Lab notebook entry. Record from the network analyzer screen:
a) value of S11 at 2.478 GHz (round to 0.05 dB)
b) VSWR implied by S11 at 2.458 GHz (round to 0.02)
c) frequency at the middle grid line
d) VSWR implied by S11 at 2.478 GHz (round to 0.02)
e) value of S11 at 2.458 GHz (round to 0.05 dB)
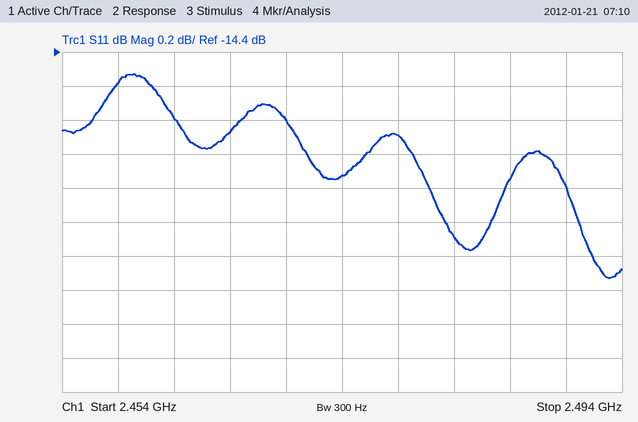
-14.90 dB
1.46
2.474 GHz
1.44
-14.60 dB
